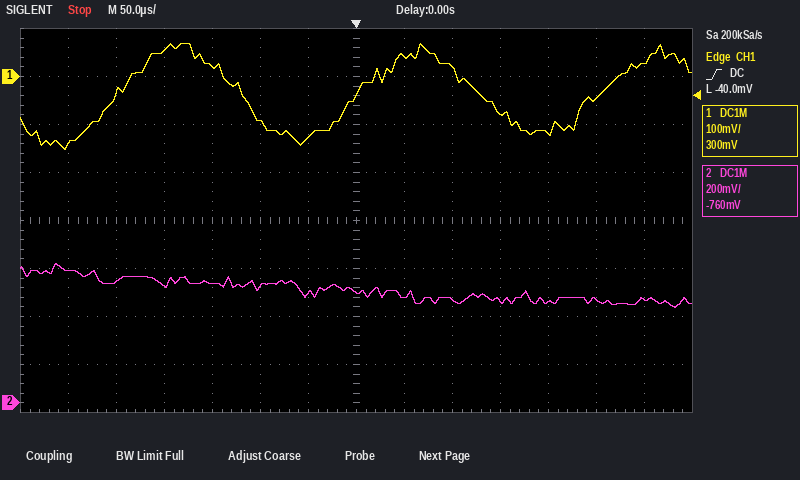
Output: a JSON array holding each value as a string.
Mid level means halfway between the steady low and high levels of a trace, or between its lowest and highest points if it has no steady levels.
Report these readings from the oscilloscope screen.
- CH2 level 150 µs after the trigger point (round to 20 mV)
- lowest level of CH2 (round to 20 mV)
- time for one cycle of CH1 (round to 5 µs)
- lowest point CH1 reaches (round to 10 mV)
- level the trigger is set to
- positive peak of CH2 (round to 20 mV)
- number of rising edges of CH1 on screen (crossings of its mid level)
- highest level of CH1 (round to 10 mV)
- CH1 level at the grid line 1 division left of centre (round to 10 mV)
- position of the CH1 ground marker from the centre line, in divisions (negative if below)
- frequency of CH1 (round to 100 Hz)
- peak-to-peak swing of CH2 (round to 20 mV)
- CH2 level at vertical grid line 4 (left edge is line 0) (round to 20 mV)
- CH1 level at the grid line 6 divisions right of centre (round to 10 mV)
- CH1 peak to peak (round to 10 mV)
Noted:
["420 mV", "400 mV", "250 µs", "-150 mV", "-40.0 mV", "580 mV", "3", "70 mV", "-130 mV", "+3.0 div", "4.0 kHz", "180 mV", "500 mV", "30 mV", "220 mV"]
